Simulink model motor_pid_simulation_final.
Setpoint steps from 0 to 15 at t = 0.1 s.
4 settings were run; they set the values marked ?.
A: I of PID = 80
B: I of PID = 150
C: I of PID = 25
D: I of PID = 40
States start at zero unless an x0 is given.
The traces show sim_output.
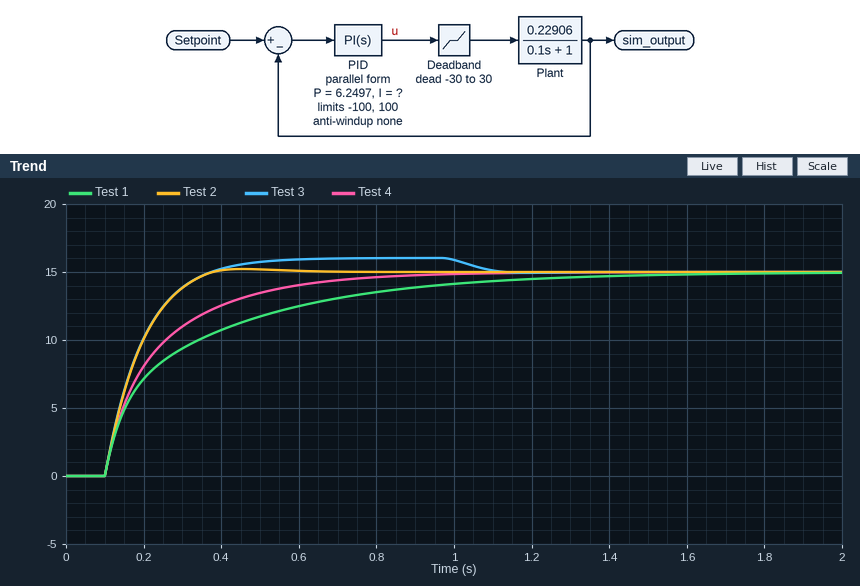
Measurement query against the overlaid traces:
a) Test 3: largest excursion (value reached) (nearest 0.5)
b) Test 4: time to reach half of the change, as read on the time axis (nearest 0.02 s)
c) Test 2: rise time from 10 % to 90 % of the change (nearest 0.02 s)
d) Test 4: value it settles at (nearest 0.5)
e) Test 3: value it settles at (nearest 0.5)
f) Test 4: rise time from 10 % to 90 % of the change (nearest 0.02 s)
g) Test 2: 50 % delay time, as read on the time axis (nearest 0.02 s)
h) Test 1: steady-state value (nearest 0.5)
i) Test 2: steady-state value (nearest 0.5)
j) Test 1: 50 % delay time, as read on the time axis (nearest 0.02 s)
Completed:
16.0
0.18 s
0.18 s
15.0
15.0
0.40 s
0.16 s
15.0
15.0
0.22 s
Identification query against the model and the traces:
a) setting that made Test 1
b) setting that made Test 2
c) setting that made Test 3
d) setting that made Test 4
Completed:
C
A
B
D
